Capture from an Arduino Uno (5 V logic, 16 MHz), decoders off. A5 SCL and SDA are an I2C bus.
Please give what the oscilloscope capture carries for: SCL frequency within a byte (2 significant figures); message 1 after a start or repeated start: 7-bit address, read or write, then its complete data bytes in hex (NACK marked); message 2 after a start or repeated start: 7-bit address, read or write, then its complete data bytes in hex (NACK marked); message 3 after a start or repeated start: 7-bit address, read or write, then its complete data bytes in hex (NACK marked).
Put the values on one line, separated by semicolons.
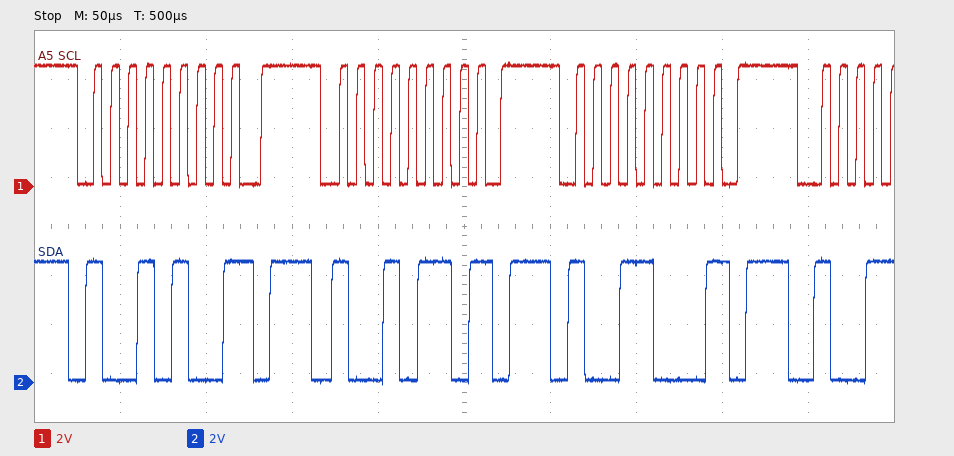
100 kHz; 0x4A write NACK; 0x4B write NACK; 0x4C write NACK
